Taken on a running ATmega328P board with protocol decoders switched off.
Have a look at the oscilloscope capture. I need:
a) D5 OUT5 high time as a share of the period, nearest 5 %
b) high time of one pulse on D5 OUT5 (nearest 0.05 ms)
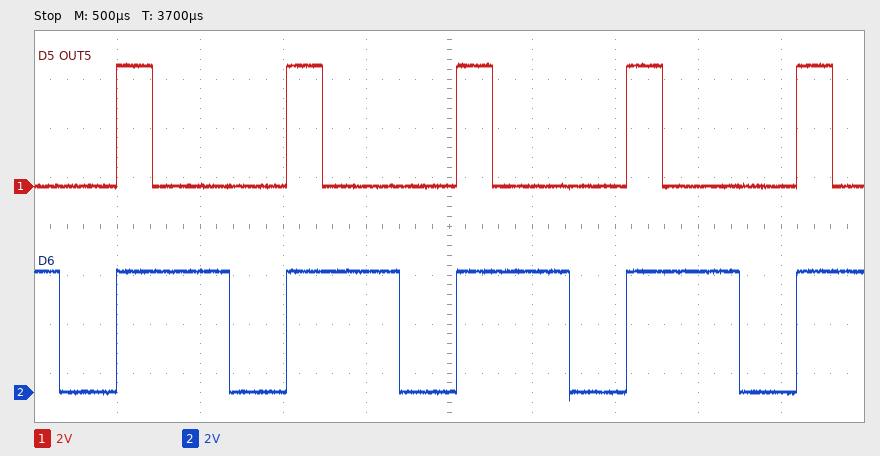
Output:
20 %
0.20 ms
